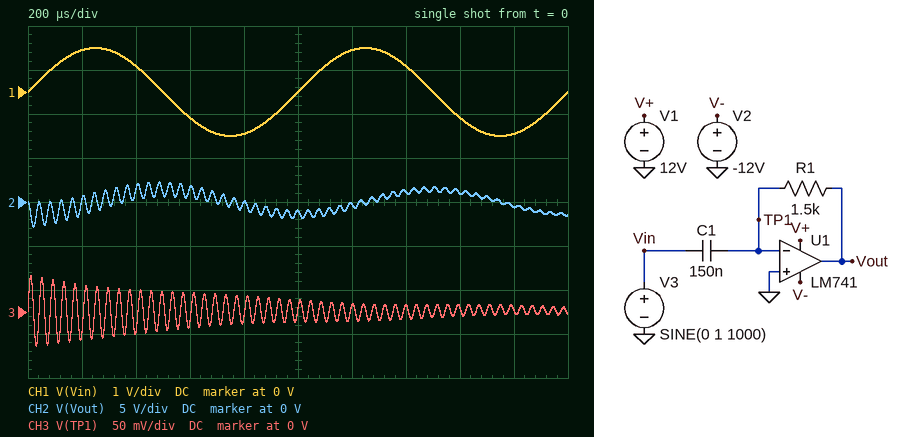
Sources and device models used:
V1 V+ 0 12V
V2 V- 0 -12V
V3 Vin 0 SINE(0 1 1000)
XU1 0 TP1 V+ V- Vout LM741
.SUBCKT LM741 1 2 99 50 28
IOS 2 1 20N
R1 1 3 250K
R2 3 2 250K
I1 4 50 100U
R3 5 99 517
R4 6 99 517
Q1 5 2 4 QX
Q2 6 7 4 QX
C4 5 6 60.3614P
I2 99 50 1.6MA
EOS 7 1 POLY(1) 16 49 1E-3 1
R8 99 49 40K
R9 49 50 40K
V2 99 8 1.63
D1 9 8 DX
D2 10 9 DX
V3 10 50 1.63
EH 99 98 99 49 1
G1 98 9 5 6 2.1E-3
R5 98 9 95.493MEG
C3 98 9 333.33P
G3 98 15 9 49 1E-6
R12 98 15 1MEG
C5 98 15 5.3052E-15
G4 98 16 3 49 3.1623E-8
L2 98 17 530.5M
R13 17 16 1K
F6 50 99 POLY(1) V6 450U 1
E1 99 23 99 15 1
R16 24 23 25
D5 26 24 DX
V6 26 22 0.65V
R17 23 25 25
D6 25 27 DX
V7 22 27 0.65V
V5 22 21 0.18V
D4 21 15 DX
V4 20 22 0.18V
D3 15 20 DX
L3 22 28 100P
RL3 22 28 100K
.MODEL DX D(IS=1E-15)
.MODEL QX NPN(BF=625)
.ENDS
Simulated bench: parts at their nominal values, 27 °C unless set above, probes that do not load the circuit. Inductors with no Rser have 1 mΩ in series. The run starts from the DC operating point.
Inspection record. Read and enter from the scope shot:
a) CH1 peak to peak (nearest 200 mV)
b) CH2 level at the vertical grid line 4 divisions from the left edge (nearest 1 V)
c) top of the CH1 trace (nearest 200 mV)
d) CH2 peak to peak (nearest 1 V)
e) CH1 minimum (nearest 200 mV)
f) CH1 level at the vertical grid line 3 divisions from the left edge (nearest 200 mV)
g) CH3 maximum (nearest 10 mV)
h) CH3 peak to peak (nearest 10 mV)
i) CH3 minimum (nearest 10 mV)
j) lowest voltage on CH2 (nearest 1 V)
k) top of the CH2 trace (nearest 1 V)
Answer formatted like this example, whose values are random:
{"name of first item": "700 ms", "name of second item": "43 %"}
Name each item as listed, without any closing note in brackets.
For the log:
{"CH1 peak to peak": "2.0 V", "CH2 level at the vertical grid line 4 divisions from the left edge": "0 V", "top of the CH1 trace": "1.0 V", "CH2 peak to peak": "5 V", "CH1 minimum": "-1.0 V", "CH1 level at the vertical grid line 3 divisions from the left edge": "-600 mV", "CH3 maximum": "40 mV", "CH3 peak to peak": "80 mV", "CH3 minimum": "-40 mV", "lowest voltage on CH2": "-3 V", "top of the CH2 trace": "2 V"}
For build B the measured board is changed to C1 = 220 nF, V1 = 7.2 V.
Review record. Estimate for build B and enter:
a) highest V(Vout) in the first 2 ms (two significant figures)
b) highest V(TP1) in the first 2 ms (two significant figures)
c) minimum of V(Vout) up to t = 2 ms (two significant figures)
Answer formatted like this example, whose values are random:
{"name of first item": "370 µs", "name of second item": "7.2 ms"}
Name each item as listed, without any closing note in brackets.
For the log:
{"highest V(Vout) in the first 2 ms": "3.5 V", "highest V(TP1) in the first 2 ms": "51 mV", "minimum of V(Vout) up to t = 2 ms": "-4.1 V"}
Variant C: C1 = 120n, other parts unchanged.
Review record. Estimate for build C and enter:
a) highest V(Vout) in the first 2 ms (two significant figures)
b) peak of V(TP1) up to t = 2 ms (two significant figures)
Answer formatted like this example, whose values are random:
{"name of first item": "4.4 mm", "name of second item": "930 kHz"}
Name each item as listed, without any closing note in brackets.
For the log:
{"highest V(Vout) in the first 2 ms": "1.7 V", "peak of V(TP1) up to t = 2 ms": "37 mV"}
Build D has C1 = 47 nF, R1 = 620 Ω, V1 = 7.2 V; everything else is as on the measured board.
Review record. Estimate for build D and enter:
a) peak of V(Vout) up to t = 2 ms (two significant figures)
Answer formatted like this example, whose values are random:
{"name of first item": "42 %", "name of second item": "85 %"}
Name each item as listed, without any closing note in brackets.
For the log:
{"peak of V(Vout) up to t = 2 ms": "190 mV"}
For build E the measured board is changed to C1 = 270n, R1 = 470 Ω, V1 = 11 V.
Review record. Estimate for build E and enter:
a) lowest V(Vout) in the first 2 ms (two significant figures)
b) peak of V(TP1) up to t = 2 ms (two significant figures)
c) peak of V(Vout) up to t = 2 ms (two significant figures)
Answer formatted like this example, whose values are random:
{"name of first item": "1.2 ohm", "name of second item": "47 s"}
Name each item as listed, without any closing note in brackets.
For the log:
{"lowest V(Vout) in the first 2 ms": "-1.6 V", "peak of V(TP1) up to t = 2 ms": "32 mV", "peak of V(Vout) up to t = 2 ms": "1.1 V"}
